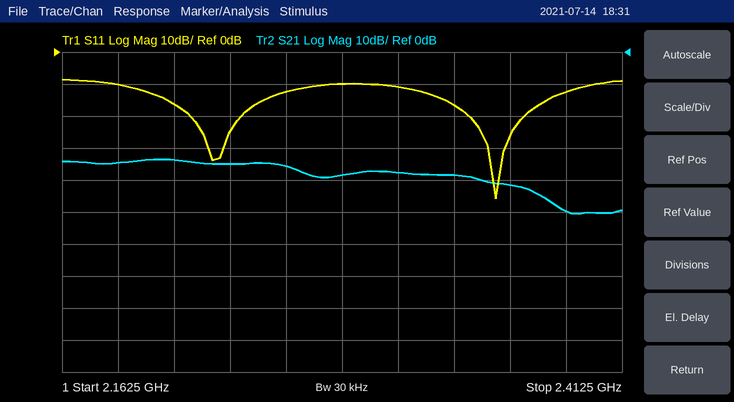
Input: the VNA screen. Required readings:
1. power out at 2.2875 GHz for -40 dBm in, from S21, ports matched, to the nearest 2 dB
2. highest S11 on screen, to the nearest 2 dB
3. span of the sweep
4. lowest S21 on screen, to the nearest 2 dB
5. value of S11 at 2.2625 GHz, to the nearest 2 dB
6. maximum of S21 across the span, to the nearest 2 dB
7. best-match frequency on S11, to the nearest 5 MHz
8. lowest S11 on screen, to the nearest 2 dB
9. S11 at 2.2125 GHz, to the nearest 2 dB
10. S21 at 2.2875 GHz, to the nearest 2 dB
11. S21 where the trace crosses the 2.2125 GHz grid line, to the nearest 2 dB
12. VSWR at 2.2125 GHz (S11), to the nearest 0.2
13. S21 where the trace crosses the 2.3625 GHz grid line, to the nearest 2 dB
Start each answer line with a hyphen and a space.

- -78 dBm
- -8 dB
- 250 MHz
- -50 dB
- -12 dB
- -34 dB
- 2.355 GHz
- -46 dB
- -16 dB
- -38 dB
- -34 dB
- 1.4
- -42 dB
